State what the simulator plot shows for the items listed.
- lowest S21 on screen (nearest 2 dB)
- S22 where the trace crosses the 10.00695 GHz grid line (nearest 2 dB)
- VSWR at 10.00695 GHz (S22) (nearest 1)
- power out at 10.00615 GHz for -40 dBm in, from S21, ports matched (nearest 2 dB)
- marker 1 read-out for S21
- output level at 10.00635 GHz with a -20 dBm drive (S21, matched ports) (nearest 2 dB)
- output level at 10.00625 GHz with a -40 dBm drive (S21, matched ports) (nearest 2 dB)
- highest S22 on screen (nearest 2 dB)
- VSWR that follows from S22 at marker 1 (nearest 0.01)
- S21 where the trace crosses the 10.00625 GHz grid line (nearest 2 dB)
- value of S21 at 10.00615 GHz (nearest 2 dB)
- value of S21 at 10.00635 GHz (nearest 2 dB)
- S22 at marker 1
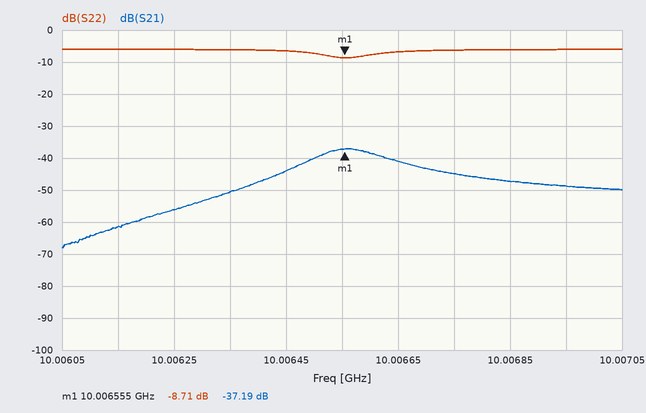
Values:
-68 dB
-6 dB
3
-102 dBm
-37.19 dB
-70 dBm
-96 dBm
-6 dB
2.16
-56 dB
-62 dB
-50 dB
-8.71 dB
